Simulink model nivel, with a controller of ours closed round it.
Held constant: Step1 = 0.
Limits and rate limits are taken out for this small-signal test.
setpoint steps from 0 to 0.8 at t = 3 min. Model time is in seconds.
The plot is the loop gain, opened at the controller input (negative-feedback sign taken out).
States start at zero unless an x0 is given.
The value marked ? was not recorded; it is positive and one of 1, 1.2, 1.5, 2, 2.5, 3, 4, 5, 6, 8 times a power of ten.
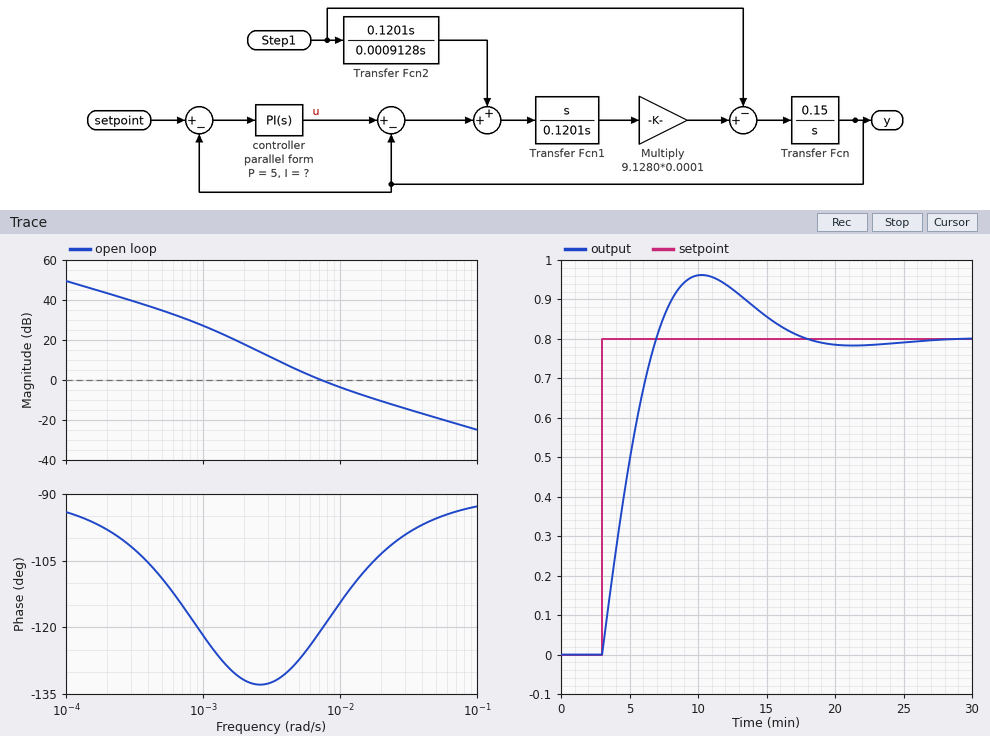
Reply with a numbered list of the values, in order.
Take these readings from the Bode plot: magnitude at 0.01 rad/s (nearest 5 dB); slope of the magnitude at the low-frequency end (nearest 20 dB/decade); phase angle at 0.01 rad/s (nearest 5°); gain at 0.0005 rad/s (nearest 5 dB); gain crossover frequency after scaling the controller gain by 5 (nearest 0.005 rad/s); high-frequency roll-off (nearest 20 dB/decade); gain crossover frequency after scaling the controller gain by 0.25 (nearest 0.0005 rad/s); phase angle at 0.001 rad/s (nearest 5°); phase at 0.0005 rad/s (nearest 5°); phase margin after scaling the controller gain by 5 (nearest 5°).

1. -5 dB
2. -20 dB/decade
3. -115°
4. 35 dB
5. 0.030 rad/s
6. -20 dB/decade
7. 0.0030 rad/s
8. -120°
9. -110°
10. 80°
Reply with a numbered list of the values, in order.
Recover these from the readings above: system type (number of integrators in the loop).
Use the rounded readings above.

1. 1
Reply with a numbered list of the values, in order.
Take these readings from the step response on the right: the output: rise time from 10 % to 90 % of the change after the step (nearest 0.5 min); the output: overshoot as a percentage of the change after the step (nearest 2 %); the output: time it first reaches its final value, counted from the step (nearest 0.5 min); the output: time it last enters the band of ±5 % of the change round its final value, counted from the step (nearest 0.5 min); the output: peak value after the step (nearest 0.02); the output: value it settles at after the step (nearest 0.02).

1. 3.0 min
2. 20 %
3. 4.0 min
4. 12.5 min
5. 0.96
6. 0.80
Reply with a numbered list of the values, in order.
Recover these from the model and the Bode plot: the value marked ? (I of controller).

1. 0.03
